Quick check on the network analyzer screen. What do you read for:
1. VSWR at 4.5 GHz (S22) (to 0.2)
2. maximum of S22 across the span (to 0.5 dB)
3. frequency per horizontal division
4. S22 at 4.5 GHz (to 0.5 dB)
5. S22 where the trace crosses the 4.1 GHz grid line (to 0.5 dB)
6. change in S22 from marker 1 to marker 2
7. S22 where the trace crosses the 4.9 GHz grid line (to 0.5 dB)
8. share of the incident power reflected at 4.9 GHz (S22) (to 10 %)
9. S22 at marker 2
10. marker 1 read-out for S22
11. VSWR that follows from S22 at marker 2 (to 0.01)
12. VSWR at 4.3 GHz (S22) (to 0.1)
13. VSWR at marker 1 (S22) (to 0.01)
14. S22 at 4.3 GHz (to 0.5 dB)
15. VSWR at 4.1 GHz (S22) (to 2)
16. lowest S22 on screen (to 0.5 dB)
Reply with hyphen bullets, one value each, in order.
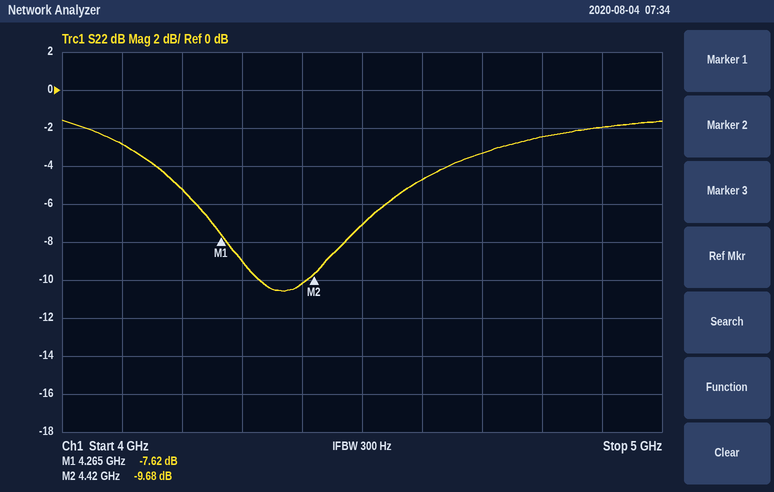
- 2.6
- -1.5 dB
- 100 MHz
- -7.0 dB
- -3.0 dB
- -2.06 dB
- -2.0 dB
- 60 %
- -9.68 dB
- -7.62 dB
- 1.98
- 2.1
- 2.42
- -9.0 dB
- 6
- -10.5 dB
